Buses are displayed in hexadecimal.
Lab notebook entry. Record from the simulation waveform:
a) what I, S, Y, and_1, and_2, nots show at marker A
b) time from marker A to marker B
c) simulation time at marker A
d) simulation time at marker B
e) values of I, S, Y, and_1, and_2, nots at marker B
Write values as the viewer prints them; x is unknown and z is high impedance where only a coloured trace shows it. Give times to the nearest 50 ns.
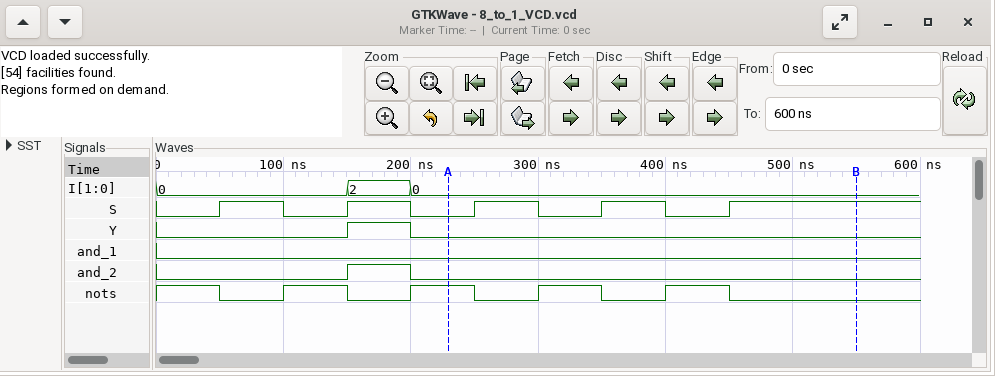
I=0, S=0, Y=0, and_1=0, and_2=0, nots=1
300 ns
250 ns
550 ns
I=0, S=1, Y=0, and_1=0, and_2=0, nots=0
